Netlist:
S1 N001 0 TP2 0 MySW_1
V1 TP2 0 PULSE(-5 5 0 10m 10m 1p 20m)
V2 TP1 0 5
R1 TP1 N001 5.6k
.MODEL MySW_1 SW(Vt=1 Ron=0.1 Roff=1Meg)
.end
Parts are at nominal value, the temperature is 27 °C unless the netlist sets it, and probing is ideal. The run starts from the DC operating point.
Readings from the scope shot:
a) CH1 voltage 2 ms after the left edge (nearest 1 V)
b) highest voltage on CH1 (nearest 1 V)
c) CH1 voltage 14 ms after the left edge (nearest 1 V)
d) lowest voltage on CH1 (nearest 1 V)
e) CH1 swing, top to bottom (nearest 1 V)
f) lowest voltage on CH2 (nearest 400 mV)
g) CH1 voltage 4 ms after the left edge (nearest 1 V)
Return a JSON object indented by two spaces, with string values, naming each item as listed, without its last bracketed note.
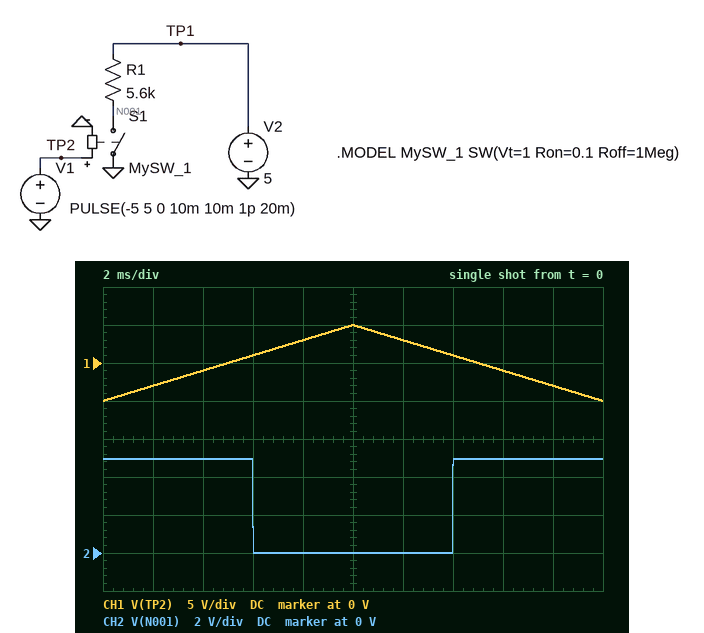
{
  "CH1 voltage 2 ms after the left edge": "-3 V",
  "highest voltage on CH1": "5 V",
  "CH1 voltage 14 ms after the left edge": "1 V",
  "lowest voltage on CH1": "-5 V",
  "CH1 swing, top to bottom": "10 V",
  "lowest voltage on CH2": "0 V",
  "CH1 voltage 4 ms after the left edge": "-1 V"
}
